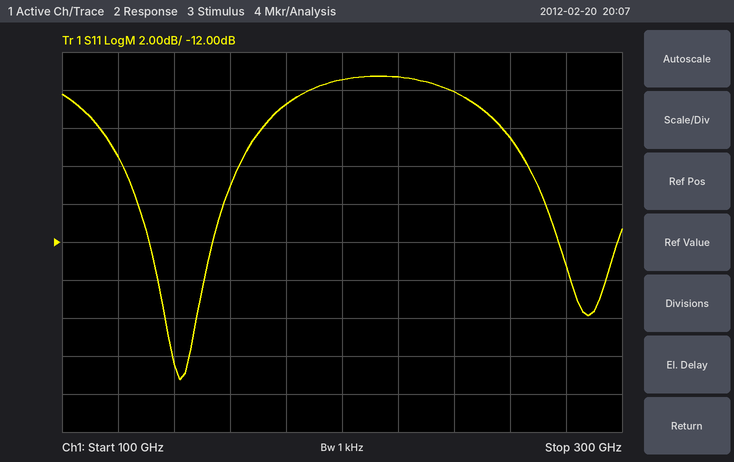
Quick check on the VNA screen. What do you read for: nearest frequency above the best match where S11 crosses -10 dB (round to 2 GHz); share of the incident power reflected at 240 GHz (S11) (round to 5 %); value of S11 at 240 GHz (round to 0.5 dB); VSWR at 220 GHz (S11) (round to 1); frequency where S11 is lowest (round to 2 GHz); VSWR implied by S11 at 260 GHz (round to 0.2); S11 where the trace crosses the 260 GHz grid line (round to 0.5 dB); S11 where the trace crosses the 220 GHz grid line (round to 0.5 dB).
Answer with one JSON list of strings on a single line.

["158 GHz", "40 %", "-4.0 dB", "5", "142 GHz", "2.8", "-6.5 dB", "-3.5 dB"]
